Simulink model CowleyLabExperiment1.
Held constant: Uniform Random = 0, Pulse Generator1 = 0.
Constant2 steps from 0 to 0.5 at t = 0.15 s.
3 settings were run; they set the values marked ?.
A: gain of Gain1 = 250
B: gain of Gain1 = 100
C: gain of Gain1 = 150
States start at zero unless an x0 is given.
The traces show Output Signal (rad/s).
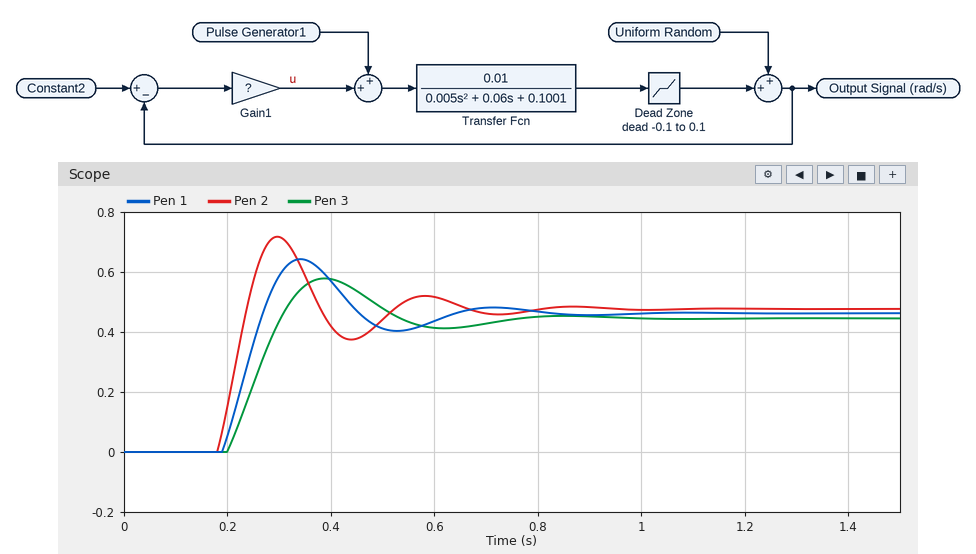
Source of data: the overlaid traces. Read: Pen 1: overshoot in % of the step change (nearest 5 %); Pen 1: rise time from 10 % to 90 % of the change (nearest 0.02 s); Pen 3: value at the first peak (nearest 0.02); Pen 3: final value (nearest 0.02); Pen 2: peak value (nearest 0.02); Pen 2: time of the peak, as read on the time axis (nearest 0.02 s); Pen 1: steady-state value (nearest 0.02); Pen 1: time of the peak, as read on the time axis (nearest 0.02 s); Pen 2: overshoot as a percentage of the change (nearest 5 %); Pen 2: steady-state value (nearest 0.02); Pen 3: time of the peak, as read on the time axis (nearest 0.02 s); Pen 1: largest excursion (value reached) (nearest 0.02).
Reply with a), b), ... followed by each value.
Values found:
a) 40 %
b) 0.06 s
c) 0.58
d) 0.44
e) 0.72
f) 0.30 s
g) 0.46
h) 0.34 s
i) 50 %
j) 0.48
k) 0.38 s
l) 0.64
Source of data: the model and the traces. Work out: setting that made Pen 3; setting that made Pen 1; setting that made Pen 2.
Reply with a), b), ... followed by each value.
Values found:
a) B
b) C
c) A
